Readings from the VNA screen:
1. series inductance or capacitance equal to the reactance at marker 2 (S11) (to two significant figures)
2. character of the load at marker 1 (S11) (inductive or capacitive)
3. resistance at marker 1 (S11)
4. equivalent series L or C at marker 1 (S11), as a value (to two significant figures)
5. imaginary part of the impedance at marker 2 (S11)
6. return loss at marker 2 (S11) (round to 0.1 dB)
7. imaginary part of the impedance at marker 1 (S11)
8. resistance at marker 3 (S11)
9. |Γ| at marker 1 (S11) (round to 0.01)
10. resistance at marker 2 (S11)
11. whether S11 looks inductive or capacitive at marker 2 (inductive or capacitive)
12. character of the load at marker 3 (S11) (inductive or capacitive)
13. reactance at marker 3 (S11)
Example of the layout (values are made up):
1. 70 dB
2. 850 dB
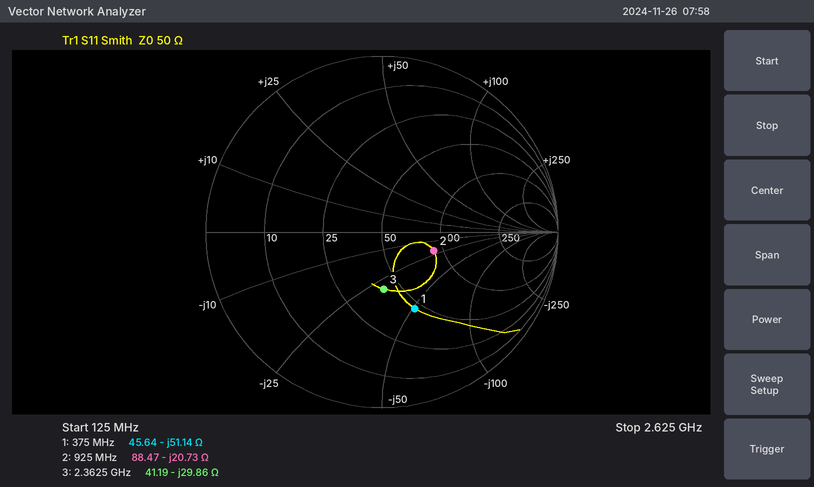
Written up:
1. 8.3 pF
2. capacitive
3. 45.64 Ω
4. 8.3 pF
5. -20.73 Ω
6. 10.1 dB
7. -51.14 Ω
8. 41.19 Ω
9. 0.47
10. 88.47 Ω
11. capacitive
12. capacitive
13. -29.86 Ω
